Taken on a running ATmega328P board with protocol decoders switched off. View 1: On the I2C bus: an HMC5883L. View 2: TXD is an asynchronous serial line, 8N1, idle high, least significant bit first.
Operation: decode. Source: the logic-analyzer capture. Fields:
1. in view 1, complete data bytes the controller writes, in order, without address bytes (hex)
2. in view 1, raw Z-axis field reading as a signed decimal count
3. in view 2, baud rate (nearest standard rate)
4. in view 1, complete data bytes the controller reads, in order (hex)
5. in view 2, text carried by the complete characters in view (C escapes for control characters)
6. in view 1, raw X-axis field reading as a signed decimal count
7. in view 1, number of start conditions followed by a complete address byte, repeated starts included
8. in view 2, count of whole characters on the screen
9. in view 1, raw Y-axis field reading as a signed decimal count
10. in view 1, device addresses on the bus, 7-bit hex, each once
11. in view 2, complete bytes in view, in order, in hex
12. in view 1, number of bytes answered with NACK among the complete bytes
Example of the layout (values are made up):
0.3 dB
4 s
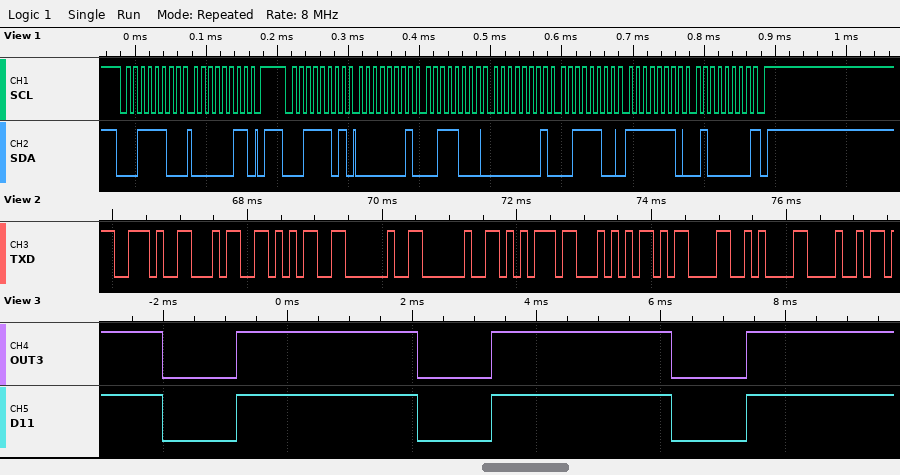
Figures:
03
316
9600 baud
01 38 01 3C FE 40
".45  uT\r\nH"
312
2
10
-448
0x1E
2E 34 35 20 20 75 54 0D 0A 48
1
